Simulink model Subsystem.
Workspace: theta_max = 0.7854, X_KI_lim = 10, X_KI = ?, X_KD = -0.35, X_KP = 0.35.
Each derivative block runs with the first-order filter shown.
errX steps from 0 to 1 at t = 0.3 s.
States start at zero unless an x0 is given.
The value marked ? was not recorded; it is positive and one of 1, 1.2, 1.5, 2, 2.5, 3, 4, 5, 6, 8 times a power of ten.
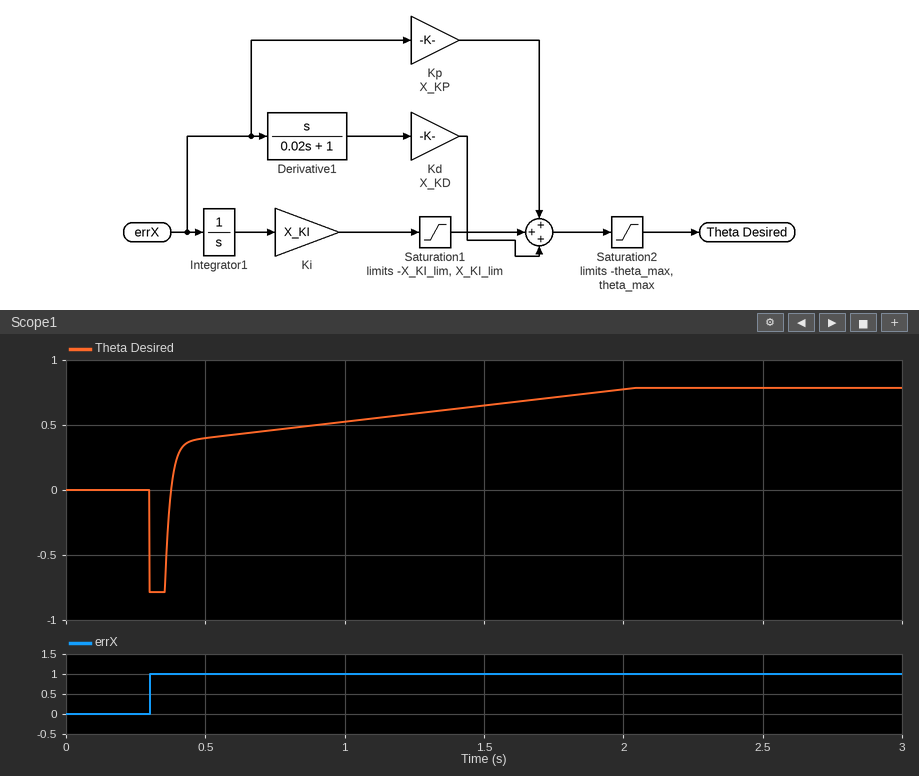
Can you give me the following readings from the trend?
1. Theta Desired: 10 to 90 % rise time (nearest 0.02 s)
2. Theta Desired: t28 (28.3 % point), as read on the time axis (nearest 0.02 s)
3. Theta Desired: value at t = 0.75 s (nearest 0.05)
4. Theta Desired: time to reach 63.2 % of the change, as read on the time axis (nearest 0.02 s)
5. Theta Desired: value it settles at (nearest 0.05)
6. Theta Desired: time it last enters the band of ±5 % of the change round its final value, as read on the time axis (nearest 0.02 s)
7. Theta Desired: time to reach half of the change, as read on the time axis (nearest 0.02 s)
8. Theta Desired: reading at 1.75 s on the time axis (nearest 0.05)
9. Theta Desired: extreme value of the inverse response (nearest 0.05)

1.34 s
0.40 s
0.45
0.88 s
0.80
1.88 s
0.48 s
0.70
-0.80
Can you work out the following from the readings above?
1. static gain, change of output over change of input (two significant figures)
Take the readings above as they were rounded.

0.80
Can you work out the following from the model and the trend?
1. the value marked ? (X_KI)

0.25
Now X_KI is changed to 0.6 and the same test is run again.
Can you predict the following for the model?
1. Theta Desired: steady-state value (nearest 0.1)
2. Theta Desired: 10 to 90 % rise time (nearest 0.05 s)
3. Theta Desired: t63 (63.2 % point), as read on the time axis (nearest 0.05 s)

0.8
0.50 s
0.55 s
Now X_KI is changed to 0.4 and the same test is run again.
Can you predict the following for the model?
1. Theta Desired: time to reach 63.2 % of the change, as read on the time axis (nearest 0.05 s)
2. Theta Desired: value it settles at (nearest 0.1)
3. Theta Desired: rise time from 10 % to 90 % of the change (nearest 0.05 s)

0.65 s
0.8
0.80 s
